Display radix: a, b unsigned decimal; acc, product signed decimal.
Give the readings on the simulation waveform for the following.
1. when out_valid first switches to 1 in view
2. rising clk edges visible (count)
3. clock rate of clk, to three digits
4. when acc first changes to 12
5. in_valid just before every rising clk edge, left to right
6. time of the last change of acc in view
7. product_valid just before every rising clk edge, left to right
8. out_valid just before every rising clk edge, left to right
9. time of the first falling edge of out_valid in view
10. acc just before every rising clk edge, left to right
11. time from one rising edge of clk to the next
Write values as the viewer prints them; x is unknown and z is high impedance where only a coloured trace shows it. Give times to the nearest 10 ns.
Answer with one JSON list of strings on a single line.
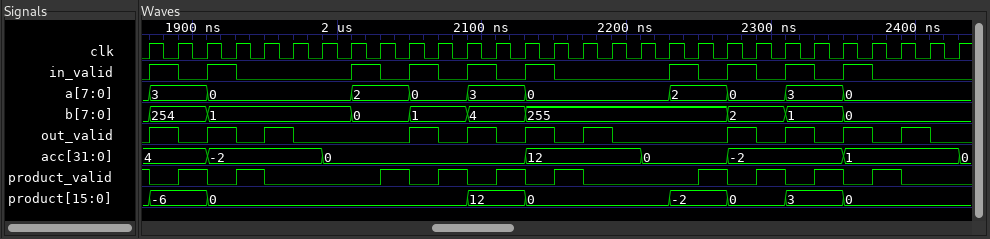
["1870 ns", "29", "50.0 MHz", "2130 ns", "0 1 0 1 0 0 0 0 1 0 1 0 1 0 1 0 0 0 0 1 0 1 0 1 0 1 0 0 0", "2430 ns", "1 0 1 0 1 0 0 0 0 1 0 1 0 1 0 1 0 0 0 0 1 0 1 0 1 0 1 0 0", "0 1 0 1 0 1 0 0 0 0 1 0 1 0 1 0 1 0 0 0 0 1 0 1 0 1 0 1 0", "1890 ns", "4, 4, 4, -2, -2, -2, -2, 0, 0, 0, 0, 0, 0, 0, 12, 12, 12, 12, 0, 0, 0, -2, -2, -2, -2, 1, 1, 1, 1", "20 ns"]
